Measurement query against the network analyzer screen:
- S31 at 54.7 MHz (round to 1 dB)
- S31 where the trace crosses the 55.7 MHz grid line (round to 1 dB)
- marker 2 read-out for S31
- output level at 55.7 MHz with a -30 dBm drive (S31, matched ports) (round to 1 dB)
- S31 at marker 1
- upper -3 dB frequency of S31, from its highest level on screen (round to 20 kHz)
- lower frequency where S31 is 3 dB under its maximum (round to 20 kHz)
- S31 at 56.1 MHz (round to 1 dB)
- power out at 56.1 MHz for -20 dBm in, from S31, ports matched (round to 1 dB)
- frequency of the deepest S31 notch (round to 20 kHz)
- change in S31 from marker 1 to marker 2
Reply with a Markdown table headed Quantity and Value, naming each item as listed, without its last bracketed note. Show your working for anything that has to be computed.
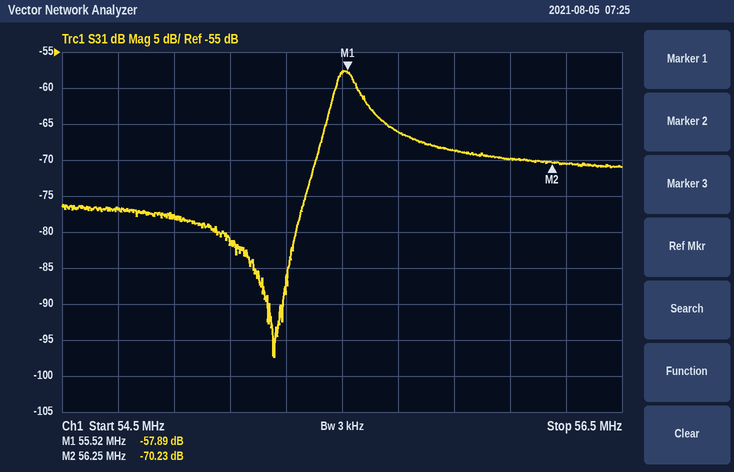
| Quantity | Value |
|---|---|
| S31 at 54.7 MHz | -77 dB |
| S31 where the trace crosses the 55.7 MHz grid line | -66 dB |
| marker 2 read-out for S31 | -70.23 dB |
| output level at 55.7 MHz with a -30 dBm drive (S31, matched ports) | -30 dBm + (-66 dB) = -96 dBm |
| S31 at marker 1 | -57.89 dB |
| upper -3 dB frequency of S31, from its highest level on screen | 55.56 MHz |
| lower frequency where S31 is 3 dB under its maximum | 55.48 MHz |
| S31 at 56.1 MHz | -70 dB |
| power out at 56.1 MHz for -20 dBm in, from S31, ports matched | -20 dBm + (-70 dB) = -90 dBm |
| frequency of the deepest S31 notch | 55.26 MHz |
| change in S31 from marker 1 to marker 2 | -70.23 − (-57.89) = -12.34 dB |
